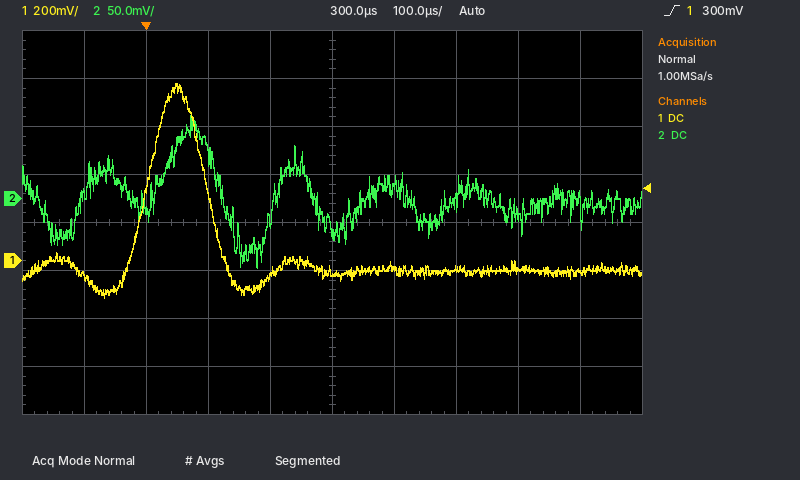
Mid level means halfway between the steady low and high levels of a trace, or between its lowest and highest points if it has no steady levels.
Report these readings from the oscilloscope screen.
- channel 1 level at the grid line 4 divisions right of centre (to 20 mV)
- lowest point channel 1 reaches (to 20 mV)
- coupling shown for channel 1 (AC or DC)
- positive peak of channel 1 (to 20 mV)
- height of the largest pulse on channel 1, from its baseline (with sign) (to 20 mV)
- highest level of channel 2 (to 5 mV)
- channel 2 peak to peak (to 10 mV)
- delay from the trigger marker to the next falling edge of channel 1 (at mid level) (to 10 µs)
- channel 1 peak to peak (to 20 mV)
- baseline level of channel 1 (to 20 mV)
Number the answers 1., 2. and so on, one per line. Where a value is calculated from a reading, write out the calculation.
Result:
1. -40 mV
2. -160 mV
3. DC
4. 740 mV
5. 740 mV − (-40 mV) = +780 mV
6. 85 mV
7. 160 mV
8. 100 µs
9. 740 mV − (-160 mV) = 900 mV
10. -40 mV
